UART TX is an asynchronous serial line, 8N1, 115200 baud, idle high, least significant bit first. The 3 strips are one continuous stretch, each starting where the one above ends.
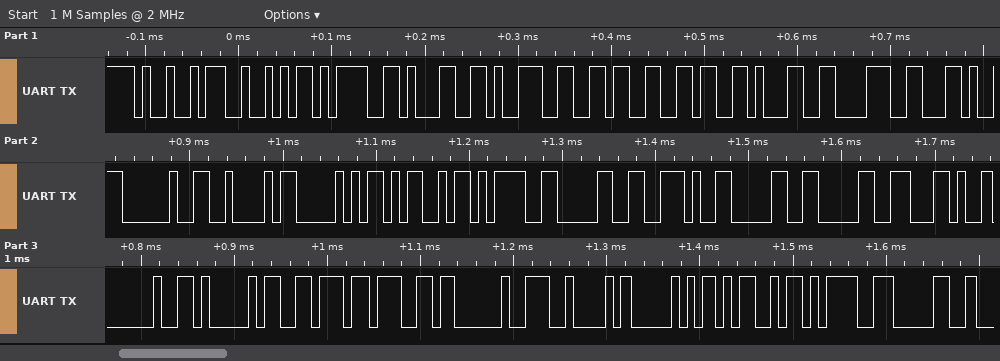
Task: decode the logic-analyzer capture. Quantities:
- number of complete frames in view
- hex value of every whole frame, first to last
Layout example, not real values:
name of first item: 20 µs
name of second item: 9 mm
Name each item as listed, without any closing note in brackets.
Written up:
number of complete frames in view: 30
hex value of every whole frame, first to last: 49 52 3D 31 39 36 36 31 38 2C 20 42 50 4D 3D 30 2E 30 30 2C 20 41 76 67 20 42 50 4D 3D 30
